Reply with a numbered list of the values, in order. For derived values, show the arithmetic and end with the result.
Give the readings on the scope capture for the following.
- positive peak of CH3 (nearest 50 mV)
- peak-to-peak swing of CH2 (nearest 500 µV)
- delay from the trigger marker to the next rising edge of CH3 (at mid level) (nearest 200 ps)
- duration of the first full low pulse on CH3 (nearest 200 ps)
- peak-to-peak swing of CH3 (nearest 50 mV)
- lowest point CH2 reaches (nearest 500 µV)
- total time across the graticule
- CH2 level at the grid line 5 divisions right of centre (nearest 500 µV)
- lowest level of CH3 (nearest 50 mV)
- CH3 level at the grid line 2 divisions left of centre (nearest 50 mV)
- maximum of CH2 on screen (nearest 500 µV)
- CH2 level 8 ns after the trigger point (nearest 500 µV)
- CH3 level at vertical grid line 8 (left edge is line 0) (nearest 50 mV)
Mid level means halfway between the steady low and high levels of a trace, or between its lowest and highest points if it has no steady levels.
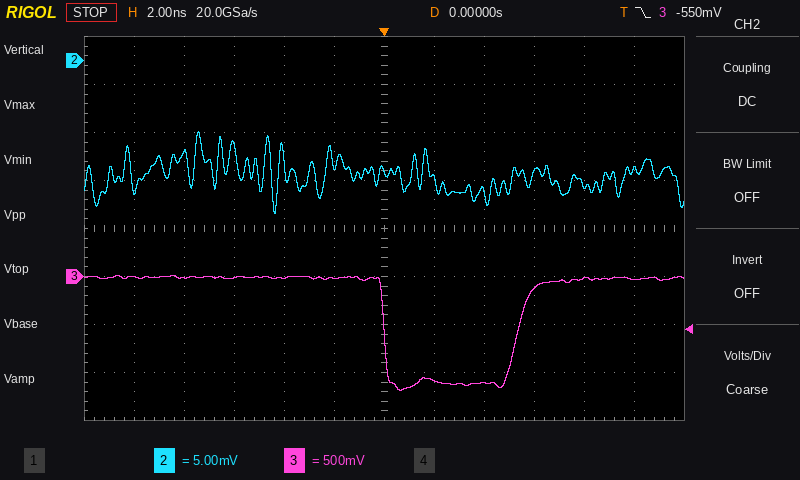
1. 0 mV
2. -7.5 mV − (-16.0 mV) = 8.5 mV
3. 5.4 ns
4. 5.4 ns
5. 0 mV − (-1.20 V) = 1.20 V
6. -16.0 mV
7. 24 ns
8. -11.5 mV
9. -1.20 V
10. 0 mV
11. -7.5 mV
12. -13.0 mV
13. -1.10 V
